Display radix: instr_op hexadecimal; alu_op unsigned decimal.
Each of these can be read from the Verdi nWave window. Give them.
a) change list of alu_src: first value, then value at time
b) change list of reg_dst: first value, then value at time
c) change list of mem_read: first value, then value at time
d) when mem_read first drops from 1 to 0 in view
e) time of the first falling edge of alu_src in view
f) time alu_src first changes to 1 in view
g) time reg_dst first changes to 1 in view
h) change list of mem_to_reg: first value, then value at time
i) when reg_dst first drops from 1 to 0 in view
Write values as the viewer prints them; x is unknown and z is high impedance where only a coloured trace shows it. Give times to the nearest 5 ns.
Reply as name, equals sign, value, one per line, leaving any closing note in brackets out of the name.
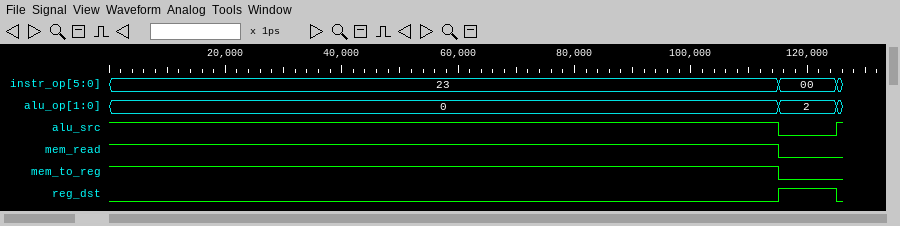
change list of alu_src: first value, then value at time = 1, 0 at 115 ns, 1 at 125 ns
change list of reg_dst: first value, then value at time = 0, 1 at 115 ns, 0 at 125 ns
change list of mem_read: first value, then value at time = 1, 0 at 115 ns
when mem_read first drops from 1 to 0 in view = 115 ns
time of the first falling edge of alu_src in view = 115 ns
time alu_src first changes to 1 in view = 125 ns
time reg_dst first changes to 1 in view = 115 ns
change list of mem_to_reg: first value, then value at time = 1, 0 at 115 ns
when reg_dst first drops from 1 to 0 in view = 125 ns
